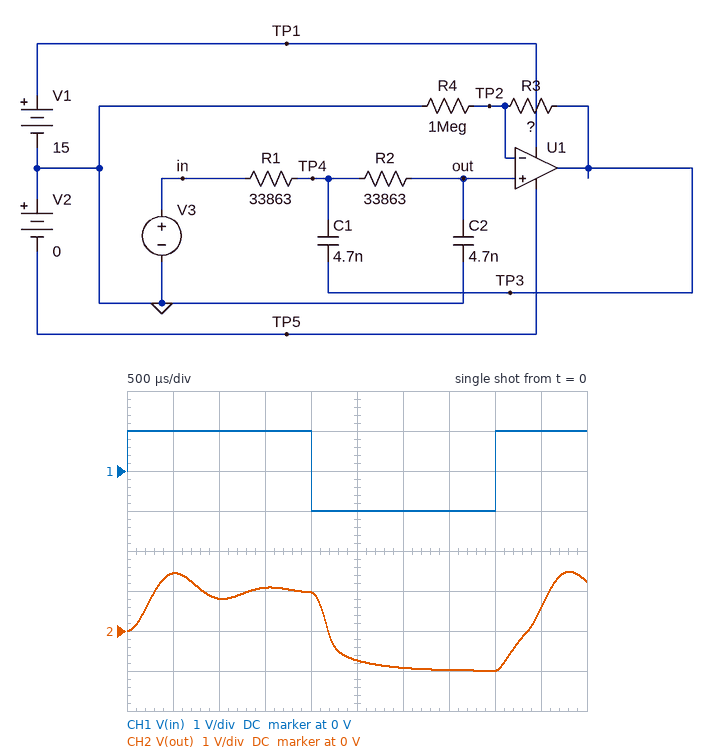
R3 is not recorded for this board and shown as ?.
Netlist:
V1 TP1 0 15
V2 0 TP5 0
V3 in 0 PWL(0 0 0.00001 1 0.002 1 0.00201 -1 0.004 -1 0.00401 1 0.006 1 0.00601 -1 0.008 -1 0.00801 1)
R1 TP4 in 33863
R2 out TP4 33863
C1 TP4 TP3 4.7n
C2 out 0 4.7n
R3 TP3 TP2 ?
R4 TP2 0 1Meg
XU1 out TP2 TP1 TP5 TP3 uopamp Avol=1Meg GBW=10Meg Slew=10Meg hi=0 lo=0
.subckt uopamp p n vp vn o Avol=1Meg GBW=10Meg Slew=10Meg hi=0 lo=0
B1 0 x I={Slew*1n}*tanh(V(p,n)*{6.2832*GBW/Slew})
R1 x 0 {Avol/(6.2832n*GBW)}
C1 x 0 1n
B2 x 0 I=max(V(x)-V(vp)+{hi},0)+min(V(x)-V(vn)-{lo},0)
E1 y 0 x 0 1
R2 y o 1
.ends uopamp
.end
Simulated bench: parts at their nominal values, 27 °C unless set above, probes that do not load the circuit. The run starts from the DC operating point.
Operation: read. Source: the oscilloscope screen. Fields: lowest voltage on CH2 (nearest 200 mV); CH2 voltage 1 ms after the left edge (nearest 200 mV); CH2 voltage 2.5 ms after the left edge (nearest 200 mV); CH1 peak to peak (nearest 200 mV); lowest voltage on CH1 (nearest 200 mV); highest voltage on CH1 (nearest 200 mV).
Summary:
-1.0 V
800 mV
-800 mV
2.0 V
-1.0 V
1.0 V
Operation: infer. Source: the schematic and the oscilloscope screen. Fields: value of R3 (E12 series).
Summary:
1.5 MΩ
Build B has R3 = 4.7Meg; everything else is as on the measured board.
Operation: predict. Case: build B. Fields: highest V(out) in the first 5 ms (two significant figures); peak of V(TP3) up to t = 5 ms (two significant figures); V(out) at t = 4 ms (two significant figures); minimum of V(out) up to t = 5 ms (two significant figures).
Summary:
4.5 V
15 V
-1.0 V
-2.9 V
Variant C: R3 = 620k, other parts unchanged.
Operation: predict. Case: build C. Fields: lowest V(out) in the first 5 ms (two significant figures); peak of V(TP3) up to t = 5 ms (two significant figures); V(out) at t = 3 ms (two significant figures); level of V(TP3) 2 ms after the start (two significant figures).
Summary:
-990 mV
1.7 V
-880 mV
1.6 V
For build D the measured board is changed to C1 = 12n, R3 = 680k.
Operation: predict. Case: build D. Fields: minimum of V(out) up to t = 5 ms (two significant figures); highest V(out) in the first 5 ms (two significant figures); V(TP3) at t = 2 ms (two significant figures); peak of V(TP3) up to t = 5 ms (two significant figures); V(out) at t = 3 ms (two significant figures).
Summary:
-970 mV
1.8 V
1.6 V
3.0 V
-860 mV
